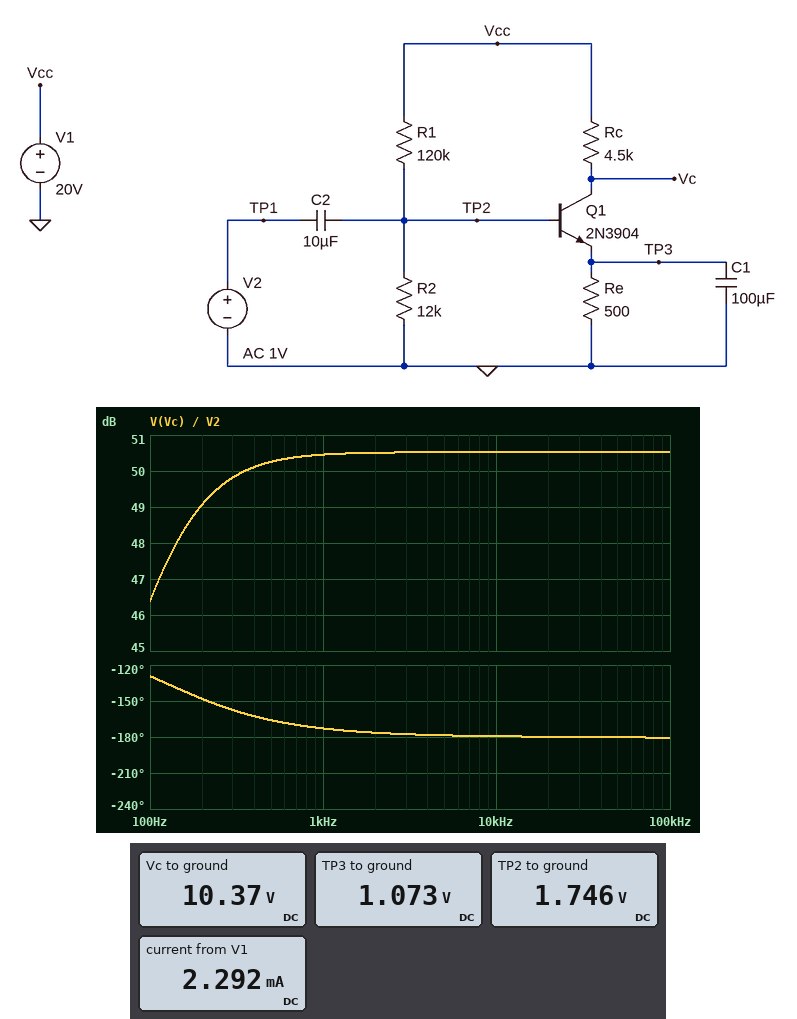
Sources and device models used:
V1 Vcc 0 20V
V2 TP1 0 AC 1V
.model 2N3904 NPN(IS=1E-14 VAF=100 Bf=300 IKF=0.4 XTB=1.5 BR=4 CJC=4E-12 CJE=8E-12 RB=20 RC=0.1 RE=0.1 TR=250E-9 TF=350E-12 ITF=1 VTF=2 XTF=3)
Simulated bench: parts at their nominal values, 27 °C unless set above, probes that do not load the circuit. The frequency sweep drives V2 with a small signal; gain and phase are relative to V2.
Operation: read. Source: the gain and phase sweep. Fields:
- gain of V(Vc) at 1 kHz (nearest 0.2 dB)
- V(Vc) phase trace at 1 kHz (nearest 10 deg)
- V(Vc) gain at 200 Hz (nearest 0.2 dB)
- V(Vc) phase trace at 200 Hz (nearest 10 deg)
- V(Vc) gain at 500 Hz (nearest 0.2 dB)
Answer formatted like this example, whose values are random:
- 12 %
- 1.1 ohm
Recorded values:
- 50.4 dB
- -170 deg
- 49.0 dB
- -150 deg
- 50.2 dB
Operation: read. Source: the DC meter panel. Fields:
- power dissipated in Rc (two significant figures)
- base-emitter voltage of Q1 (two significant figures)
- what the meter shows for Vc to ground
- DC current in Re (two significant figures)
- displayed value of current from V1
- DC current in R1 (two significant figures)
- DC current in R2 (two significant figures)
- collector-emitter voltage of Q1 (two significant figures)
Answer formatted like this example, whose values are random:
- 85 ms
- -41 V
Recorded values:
- 21 mW
- 670 mV
- 10.37 V
- 2.1 mA
- 2.292 mA
- 150 µA
- 150 µA
- 9.3 V
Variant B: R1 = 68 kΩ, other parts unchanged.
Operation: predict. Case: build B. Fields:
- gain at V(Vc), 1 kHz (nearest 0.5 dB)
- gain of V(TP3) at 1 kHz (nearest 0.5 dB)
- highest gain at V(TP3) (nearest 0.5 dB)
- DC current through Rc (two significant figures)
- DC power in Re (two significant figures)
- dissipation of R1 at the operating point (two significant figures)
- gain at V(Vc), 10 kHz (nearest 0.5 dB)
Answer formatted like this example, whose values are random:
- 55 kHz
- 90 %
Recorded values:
- 28.5 dB
- -28.5 dB
- -18.5 dB
- 4.0 mA
- 8.0 mW
- 4.4 mW
- 29.0 dB
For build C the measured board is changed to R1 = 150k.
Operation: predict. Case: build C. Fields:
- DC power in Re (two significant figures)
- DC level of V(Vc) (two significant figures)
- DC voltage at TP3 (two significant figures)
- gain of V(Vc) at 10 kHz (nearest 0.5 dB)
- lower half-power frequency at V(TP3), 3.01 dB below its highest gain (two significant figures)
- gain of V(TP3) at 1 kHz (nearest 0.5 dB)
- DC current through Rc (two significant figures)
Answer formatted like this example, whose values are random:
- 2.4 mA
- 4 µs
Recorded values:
- 1.2 mW
- 13 V
- 770 mV
- 48.0 dB
- 1.4 Hz
- -21.0 dB
- 1.5 mA
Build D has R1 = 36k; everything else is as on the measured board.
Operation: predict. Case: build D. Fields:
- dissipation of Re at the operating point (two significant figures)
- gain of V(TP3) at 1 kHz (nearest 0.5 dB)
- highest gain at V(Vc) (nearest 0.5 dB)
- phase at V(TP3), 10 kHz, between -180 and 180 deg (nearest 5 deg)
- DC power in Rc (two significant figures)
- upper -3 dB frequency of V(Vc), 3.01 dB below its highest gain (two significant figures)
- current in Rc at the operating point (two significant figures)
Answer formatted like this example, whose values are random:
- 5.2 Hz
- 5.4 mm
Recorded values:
- 8.9 mW
- -29.5 dB
- 5.5 dB
- -85 deg
- 71 mW
- 290 kHz
- 4.0 mA
